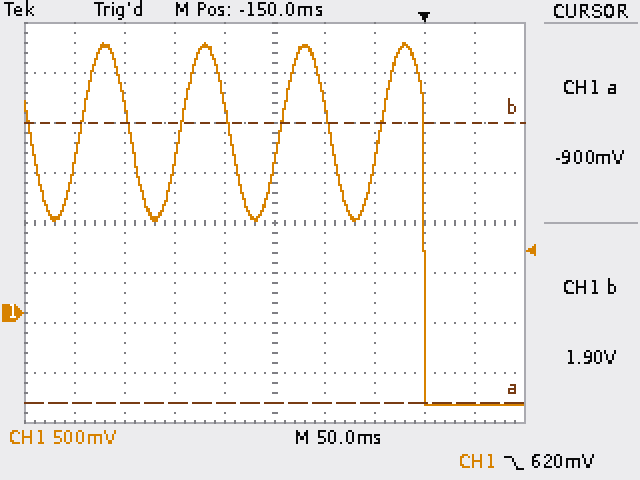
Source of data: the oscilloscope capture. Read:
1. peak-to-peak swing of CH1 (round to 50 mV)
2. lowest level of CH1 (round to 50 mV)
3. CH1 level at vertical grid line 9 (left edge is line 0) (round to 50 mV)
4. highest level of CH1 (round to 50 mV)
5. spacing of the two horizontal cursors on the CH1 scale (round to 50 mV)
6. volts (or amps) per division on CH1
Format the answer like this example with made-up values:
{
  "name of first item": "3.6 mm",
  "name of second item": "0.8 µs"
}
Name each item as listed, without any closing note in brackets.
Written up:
{
  "peak-to-peak swing of CH1": "3.60 V",
  "lowest level of CH1": "-900 mV",
  "CH1 level at vertical grid line 9 (left edge is line 0)": "-900 mV",
  "highest level of CH1": "2.70 V",
  "spacing of the two horizontal cursors on the CH1 scale": "2.80 V",
  "volts (or amps) per division on CH1": "500 mV"
}
